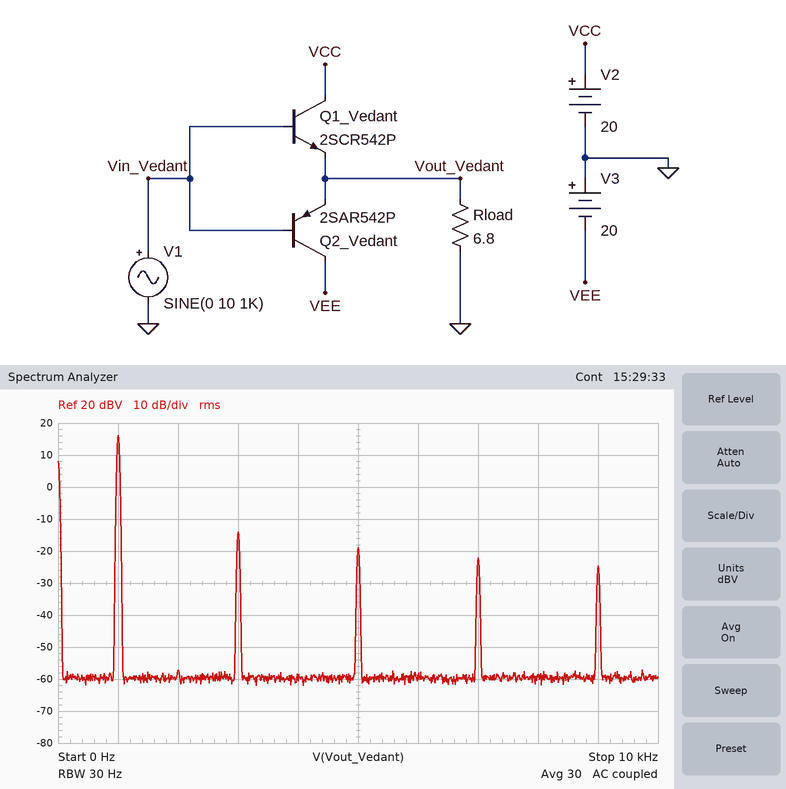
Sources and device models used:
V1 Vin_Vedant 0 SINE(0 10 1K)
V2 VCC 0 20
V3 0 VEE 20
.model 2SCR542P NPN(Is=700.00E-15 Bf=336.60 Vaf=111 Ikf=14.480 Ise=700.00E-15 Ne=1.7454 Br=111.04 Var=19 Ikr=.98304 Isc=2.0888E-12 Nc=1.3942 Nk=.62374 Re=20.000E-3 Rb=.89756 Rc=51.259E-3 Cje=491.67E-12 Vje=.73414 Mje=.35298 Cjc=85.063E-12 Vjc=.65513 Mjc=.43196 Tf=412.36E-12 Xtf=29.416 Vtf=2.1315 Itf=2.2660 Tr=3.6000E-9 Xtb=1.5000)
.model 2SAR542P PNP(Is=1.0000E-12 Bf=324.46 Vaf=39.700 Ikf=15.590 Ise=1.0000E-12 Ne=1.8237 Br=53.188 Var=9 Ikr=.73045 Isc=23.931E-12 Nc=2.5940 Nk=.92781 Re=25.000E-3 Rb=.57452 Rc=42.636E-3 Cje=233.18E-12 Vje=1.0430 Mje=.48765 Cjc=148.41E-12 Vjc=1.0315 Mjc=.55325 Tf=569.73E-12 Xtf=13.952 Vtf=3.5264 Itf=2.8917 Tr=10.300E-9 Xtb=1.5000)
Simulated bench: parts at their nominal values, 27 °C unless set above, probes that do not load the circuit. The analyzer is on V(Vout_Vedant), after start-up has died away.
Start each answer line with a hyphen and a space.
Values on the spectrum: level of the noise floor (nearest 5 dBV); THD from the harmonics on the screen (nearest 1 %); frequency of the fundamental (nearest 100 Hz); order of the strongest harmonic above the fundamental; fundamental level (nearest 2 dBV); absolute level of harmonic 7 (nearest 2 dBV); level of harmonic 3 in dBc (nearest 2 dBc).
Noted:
- -60 dBV
- 4 %
- 1.0 kHz
- 3
- 16 dBV
- -22 dBV
- -30 dBc
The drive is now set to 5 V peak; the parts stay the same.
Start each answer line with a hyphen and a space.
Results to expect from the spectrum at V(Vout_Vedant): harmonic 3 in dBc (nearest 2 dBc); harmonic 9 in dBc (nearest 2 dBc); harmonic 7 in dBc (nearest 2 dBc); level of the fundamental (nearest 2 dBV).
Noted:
- -24 dBc
- -36 dBc
- -32 dBc
- 10 dBV
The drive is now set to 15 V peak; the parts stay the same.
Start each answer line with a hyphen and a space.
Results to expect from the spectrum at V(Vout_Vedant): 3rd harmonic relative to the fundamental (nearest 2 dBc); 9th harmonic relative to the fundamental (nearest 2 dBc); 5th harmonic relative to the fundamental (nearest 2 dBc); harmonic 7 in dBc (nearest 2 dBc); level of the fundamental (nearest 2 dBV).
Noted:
- -34 dBc
- -44 dBc
- -38 dBc
- -42 dBc
- 20 dBV
